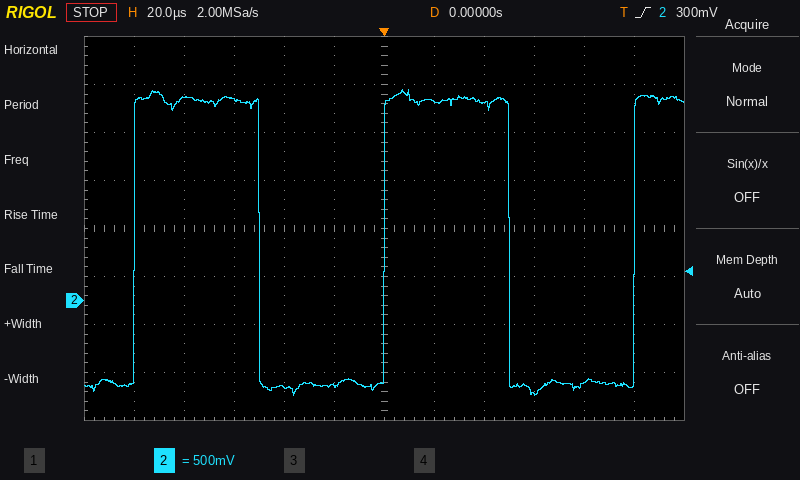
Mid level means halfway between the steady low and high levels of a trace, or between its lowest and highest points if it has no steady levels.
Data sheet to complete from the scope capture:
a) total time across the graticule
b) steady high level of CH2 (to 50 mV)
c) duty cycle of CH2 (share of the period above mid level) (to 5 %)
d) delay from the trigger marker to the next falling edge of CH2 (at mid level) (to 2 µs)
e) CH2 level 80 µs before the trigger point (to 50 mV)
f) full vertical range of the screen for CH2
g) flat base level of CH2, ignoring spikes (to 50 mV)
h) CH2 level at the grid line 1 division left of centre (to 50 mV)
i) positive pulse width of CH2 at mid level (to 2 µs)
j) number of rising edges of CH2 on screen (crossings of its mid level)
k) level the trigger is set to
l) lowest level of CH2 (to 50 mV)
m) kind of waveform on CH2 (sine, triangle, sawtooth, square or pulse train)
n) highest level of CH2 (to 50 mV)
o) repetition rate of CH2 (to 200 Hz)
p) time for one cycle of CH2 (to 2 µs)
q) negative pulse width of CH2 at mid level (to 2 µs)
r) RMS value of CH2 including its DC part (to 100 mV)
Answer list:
240 µs
2.10 V
50 %
50 µs
2.10 V
4 V
-900 mV
-900 mV
50 µs
3
300 mV
-1.00 V
square
2.20 V
10.0 kHz
100 µs
50 µs
1.6 V
